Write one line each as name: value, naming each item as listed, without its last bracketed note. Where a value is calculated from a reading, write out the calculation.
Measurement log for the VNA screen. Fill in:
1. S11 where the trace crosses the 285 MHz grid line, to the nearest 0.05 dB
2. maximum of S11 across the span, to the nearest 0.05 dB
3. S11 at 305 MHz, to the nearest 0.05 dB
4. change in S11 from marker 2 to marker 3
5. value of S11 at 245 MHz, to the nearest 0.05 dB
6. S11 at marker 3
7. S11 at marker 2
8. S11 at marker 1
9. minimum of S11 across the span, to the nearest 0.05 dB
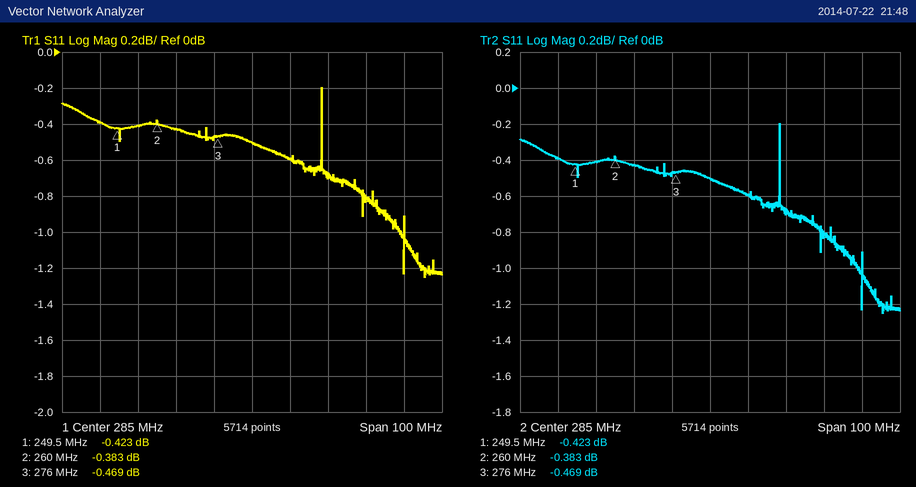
S11 where the trace crosses the 285 MHz grid line, to the nearest 0.05 dB: -0.50 dB
maximum of S11 across the span, to the nearest 0.05 dB: -0.20 dB
S11 at 305 MHz, to the nearest 0.05 dB: -0.70 dB
change in S11 from marker 2 to marker 3: -0.469 − (-0.383) = -0.086 dB
value of S11 at 245 MHz, to the nearest 0.05 dB: -0.40 dB
S11 at marker 3: -0.469 dB
S11 at marker 2: -0.383 dB
S11 at marker 1: -0.423 dB
minimum of S11 across the span, to the nearest 0.05 dB: -1.25 dB
